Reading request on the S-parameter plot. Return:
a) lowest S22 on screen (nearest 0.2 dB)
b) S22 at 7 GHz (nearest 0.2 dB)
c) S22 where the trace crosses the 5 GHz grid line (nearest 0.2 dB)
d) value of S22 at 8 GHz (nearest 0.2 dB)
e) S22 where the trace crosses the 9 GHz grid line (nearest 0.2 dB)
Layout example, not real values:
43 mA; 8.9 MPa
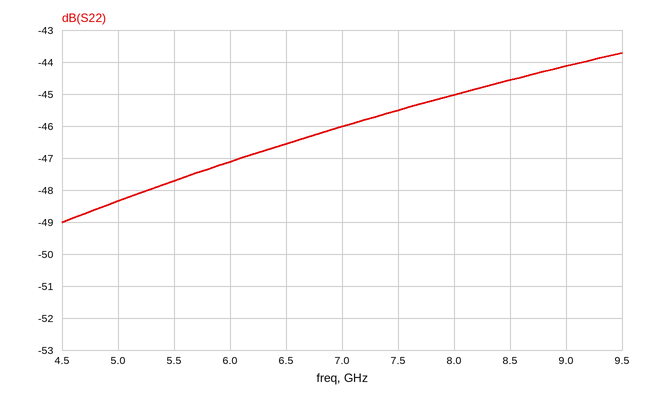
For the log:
-49.0 dB; -46.0 dB; -48.4 dB; -45.0 dB; -44.2 dB
